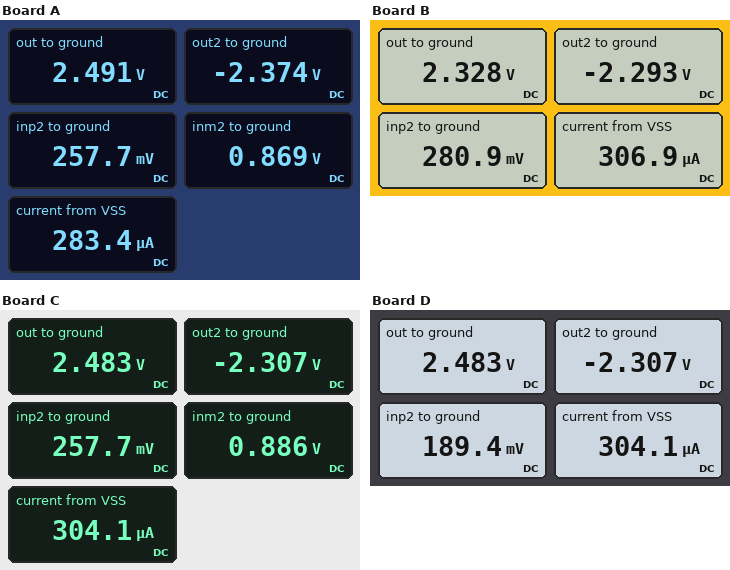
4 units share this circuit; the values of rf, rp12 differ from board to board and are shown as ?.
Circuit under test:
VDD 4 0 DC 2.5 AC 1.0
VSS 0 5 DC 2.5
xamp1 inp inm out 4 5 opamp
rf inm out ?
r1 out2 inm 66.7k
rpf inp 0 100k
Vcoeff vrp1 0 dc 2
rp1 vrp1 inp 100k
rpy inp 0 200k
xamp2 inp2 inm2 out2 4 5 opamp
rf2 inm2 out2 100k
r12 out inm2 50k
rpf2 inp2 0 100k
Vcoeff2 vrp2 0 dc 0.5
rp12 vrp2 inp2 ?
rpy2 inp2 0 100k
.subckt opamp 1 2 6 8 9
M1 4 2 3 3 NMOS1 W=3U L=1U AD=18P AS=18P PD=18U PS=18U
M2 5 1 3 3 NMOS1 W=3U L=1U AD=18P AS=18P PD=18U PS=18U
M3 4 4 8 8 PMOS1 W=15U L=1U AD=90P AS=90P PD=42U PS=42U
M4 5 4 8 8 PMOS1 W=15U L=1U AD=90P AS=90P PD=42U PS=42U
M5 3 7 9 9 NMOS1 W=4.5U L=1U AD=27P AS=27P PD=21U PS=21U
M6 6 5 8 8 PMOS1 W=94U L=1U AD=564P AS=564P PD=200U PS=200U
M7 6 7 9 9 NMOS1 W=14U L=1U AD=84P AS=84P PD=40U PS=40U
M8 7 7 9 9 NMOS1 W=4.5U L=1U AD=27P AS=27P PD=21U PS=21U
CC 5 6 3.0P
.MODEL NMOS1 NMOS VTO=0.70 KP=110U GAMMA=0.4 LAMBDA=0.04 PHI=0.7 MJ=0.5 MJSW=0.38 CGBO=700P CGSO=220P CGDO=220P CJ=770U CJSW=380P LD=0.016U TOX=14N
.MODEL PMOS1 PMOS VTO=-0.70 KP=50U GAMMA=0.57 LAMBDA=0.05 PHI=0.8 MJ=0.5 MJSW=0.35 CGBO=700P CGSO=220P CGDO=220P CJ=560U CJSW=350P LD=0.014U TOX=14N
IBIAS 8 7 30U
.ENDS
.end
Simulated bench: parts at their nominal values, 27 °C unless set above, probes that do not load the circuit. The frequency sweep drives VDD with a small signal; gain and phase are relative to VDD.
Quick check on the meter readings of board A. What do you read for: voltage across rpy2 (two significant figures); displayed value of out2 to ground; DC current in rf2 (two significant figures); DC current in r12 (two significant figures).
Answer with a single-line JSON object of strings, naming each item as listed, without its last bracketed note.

{"voltage across rpy2": "260 mV", "displayed value of out2 to ground": "-2.374 V", "DC current in rf2": "32 µA", "DC current in r12": "32 µA"}
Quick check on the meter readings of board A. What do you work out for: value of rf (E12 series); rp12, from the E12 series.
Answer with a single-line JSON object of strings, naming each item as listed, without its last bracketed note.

{"value of rf": "150 kΩ", "rp12, from the E12 series": "47 kΩ"}
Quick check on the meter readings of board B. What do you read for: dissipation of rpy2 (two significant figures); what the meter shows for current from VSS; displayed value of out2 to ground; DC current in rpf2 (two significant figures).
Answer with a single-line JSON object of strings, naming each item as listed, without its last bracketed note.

{"dissipation of rpy2": "790 nW", "what the meter shows for current from VSS": "306.9 µA", "displayed value of out2 to ground": "-2.293 V", "DC current in rpf2": "2.8 µA"}
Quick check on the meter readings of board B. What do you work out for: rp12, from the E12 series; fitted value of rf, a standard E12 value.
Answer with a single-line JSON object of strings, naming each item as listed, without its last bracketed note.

{"rp12, from the E12 series": "39 kΩ", "fitted value of rf, a standard E12 value": "33 kΩ"}
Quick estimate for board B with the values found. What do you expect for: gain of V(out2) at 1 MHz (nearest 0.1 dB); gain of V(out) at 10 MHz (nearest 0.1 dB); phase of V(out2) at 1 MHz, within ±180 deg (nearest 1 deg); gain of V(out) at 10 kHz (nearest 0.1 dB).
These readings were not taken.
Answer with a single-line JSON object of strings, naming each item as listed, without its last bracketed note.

{"gain of V(out2) at 1 MHz": "-18.8 dB", "gain of V(out) at 10 MHz": "0.2 dB", "phase of V(out2) at 1 MHz, within ±180 deg": "75 deg", "gain of V(out) at 10 kHz": "-36.6 dB"}
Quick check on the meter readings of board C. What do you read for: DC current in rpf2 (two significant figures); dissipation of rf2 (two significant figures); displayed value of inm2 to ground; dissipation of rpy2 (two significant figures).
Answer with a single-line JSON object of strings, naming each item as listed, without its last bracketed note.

{"DC current in rpf2": "2.6 µA", "dissipation of rf2": "100 µW", "displayed value of inm2 to ground": "0.886 V", "dissipation of rpy2": "660 nW"}
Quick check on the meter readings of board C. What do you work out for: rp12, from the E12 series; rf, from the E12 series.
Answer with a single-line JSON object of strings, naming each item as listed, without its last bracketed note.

{"rp12, from the E12 series": "47 kΩ", "rf, from the E12 series": "47 kΩ"}
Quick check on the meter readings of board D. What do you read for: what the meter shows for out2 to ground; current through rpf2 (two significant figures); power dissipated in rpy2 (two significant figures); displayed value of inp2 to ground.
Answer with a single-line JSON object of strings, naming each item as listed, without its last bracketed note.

{"what the meter shows for out2 to ground": "-2.307 V", "current through rpf2": "1.9 µA", "power dissipated in rpy2": "360 nW", "displayed value of inp2 to ground": "189.4 mV"}
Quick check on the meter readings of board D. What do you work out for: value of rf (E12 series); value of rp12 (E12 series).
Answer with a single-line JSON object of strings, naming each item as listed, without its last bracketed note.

{"value of rf": "47 kΩ", "value of rp12": "82 kΩ"}
